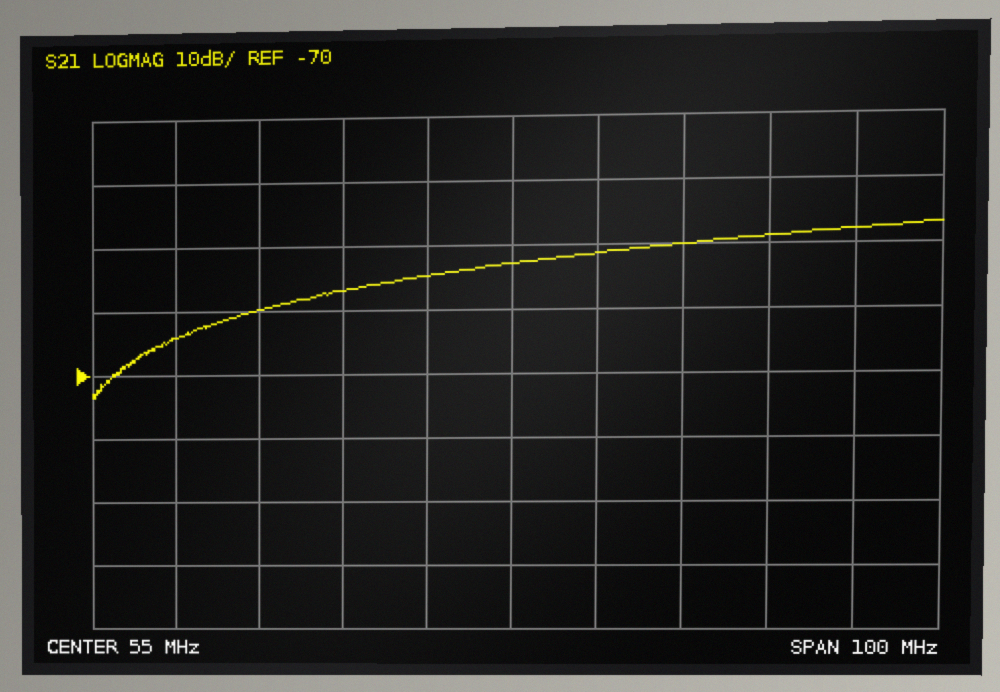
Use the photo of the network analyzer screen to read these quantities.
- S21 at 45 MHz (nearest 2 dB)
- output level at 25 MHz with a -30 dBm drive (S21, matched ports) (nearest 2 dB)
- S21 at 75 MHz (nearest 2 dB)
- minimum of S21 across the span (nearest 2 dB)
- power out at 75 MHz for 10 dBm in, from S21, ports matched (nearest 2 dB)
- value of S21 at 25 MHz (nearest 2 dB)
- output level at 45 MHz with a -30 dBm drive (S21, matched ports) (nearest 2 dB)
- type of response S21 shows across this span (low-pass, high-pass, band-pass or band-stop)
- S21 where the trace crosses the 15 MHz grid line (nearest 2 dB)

-54 dB
-90 dBm
-50 dB
-74 dB
-40 dBm
-60 dB
-84 dBm
high-pass
-64 dB
